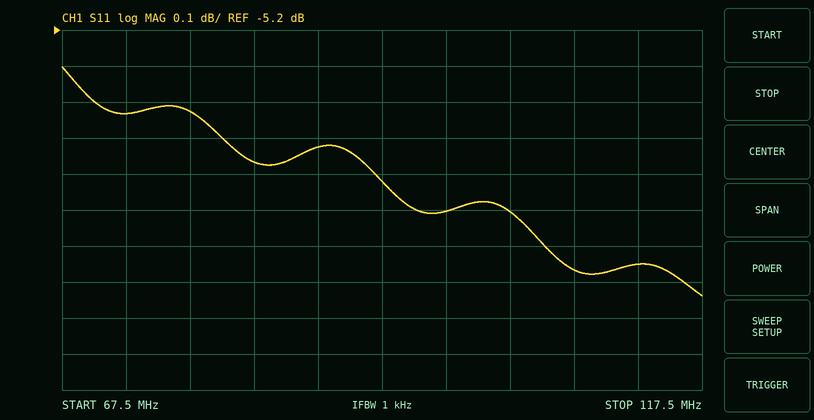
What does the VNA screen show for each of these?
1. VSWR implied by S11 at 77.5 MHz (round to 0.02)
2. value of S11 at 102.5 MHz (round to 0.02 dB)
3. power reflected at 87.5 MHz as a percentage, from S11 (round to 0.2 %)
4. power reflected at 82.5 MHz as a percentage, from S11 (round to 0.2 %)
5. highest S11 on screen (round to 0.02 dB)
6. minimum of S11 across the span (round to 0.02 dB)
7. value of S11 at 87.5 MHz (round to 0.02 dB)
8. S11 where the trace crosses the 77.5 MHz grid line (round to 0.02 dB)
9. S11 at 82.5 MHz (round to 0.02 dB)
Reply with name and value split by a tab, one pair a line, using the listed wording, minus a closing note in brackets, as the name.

VSWR implied by S11 at 77.5 MHz	3.30
value of S11 at 102.5 MHz	-5.70 dB
power reflected at 87.5 MHz as a percentage, from S11	28.0 %
power reflected at 82.5 MHz as a percentage, from S11	27.8 %
highest S11 on screen	-5.30 dB
minimum of S11 across the span	-5.94 dB
value of S11 at 87.5 MHz	-5.52 dB
S11 where the trace crosses the 77.5 MHz grid line	-5.42 dB
S11 at 82.5 MHz	-5.56 dB
